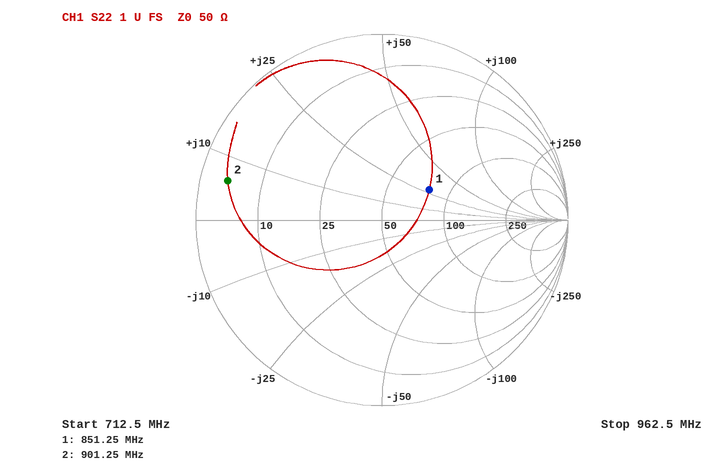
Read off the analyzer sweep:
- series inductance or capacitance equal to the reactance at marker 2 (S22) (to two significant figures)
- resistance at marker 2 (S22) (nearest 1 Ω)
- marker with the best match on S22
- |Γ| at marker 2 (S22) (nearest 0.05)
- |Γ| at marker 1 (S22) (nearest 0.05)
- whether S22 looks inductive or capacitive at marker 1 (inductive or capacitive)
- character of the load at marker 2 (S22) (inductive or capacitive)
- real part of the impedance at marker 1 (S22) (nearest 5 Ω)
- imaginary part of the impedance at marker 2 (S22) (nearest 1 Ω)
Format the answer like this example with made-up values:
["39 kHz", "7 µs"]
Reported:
["1.1 nH", "4 Ω", "marker 1", "0.85", "0.30", "inductive", "inductive", "80 Ω", "+6 Ω"]
